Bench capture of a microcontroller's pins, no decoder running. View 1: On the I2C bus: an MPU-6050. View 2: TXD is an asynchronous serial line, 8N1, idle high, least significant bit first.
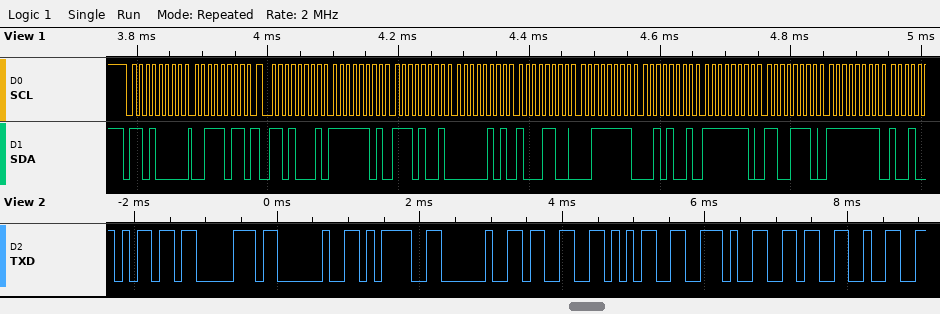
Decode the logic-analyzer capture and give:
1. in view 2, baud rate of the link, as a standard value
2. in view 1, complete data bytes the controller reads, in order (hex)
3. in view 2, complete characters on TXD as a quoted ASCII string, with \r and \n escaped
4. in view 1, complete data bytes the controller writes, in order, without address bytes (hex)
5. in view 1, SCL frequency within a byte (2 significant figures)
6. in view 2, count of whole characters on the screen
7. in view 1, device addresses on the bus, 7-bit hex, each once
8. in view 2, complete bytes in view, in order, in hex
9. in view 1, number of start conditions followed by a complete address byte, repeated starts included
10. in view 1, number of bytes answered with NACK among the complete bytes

9600 baud
FD E9 05 8C 3F 29 FE CE FF
"mp = 35.62"
3B
100 kHz
10
0x68
6D 70 20 3D 20 33 35 2E 36 32
2
0
